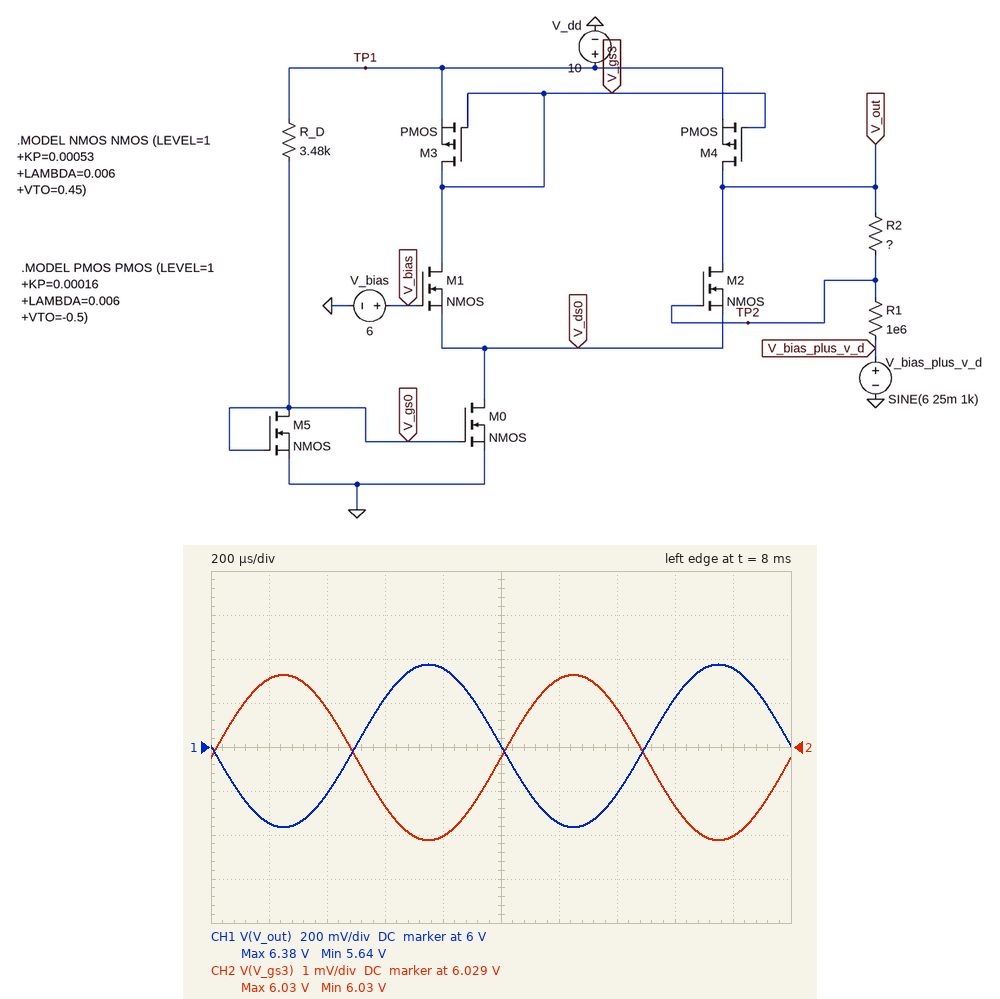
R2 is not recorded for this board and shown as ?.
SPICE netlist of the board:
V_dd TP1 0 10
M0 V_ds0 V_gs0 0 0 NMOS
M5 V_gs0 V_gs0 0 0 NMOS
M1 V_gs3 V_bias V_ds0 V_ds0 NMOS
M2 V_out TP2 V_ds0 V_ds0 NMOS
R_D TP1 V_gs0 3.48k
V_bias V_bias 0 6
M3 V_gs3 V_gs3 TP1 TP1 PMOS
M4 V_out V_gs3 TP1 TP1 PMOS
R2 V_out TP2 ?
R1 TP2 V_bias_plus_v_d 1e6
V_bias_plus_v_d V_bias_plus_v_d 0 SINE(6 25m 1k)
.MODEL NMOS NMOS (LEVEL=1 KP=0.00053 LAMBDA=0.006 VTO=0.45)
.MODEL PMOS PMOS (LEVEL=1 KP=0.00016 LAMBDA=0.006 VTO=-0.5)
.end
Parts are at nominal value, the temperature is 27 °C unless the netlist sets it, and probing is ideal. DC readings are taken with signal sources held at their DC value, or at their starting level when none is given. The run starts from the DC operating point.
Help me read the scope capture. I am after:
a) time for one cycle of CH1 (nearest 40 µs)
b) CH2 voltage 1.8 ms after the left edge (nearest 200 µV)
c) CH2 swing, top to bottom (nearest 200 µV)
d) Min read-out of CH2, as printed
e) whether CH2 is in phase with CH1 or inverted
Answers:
1.00 ms
6.0270 V
3.8 mV
6.03 V
inverted
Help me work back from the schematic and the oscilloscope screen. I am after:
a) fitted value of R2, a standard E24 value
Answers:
18 MΩ
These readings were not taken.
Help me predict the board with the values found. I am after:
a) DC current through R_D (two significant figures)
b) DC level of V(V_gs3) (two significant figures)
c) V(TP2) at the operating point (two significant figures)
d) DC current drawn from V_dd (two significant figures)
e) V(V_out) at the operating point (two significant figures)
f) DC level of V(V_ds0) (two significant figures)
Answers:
2.0 mA
6.0 V
6.0 V
3.9 mA
6.0 V
3.6 V
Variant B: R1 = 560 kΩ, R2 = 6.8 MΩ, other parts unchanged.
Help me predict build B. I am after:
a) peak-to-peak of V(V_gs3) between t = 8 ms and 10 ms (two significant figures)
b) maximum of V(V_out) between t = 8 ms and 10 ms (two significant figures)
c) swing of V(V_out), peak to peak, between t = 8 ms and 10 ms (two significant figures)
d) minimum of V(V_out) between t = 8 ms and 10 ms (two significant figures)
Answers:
2.7 mV
6.3 V
530 mV
5.7 V
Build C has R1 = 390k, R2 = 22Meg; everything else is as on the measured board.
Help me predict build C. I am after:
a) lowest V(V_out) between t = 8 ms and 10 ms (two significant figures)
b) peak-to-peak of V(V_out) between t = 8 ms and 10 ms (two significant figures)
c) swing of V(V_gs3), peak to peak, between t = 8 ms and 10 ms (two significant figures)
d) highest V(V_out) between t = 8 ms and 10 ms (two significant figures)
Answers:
5.4 V
1.3 V
10 mV
6.7 V
